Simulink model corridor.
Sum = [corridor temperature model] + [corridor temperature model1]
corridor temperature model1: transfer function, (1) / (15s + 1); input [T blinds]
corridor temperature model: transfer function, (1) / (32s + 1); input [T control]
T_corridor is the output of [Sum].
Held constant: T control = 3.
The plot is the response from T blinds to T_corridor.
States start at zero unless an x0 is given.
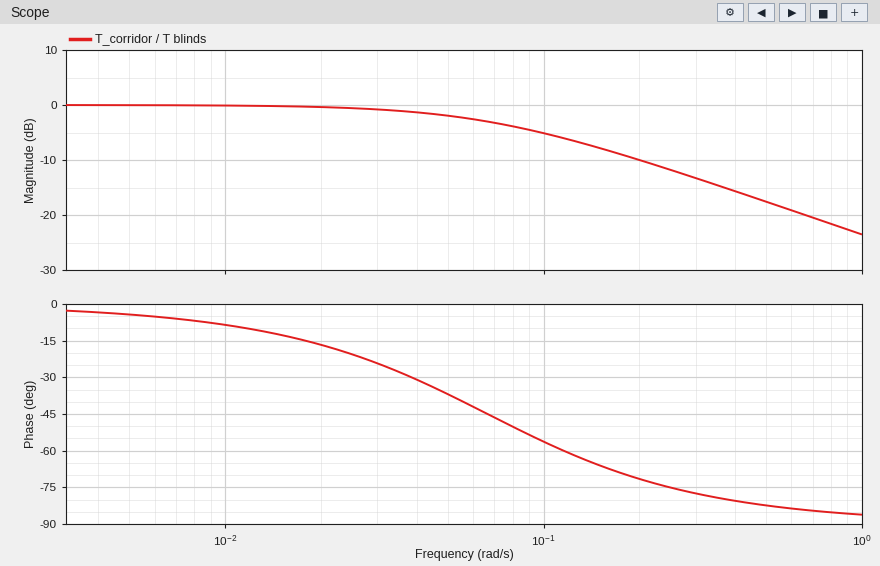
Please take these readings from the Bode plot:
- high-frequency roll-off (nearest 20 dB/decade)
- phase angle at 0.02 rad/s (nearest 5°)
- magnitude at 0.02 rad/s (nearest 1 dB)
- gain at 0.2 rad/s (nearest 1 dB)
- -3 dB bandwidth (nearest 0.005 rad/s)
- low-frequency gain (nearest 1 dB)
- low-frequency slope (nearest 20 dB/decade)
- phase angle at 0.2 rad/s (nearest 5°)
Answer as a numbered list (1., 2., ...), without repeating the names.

1. -20 dB/decade
2. -15°
3. 0 dB
4. -10 dB
5. 0.065 rad/s
6. 0 dB
7. 0 dB/decade
8. -70°
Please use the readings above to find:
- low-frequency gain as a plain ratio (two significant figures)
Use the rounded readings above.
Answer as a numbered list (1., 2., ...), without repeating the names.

1. 1.0
